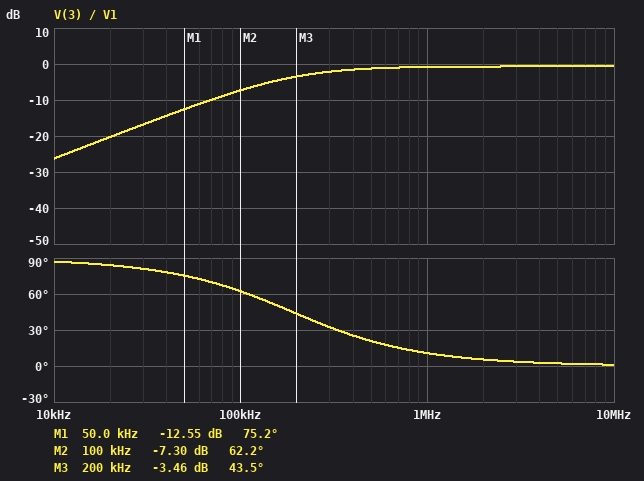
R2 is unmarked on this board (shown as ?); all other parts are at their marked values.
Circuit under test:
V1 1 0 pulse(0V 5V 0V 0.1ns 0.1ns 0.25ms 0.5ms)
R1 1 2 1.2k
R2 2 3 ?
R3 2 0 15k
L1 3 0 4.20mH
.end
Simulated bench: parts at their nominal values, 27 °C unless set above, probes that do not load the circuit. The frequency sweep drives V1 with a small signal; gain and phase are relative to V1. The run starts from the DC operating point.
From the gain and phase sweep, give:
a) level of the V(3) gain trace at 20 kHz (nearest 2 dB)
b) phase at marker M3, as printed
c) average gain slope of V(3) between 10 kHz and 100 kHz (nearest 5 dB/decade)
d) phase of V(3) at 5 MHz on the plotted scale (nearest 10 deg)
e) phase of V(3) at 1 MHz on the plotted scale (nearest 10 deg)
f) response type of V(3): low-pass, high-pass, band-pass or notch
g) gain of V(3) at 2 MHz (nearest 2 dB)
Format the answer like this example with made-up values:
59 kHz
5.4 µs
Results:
-20 dB
43.5 deg
20 dB/decade
0 deg
10 deg
high-pass
0 dB
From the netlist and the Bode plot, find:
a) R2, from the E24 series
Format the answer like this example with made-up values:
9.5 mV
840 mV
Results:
3.9 kΩ
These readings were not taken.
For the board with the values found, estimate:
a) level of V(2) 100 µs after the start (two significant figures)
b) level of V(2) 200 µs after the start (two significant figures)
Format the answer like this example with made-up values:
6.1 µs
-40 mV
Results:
3.6 V
3.6 V
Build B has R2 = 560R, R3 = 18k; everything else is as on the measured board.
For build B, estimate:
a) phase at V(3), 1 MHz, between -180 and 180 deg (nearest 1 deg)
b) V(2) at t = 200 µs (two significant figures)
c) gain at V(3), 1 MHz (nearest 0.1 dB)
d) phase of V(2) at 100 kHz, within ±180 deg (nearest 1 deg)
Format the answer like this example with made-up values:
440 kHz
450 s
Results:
4 deg
1.6 V
-0.6 dB
21 deg
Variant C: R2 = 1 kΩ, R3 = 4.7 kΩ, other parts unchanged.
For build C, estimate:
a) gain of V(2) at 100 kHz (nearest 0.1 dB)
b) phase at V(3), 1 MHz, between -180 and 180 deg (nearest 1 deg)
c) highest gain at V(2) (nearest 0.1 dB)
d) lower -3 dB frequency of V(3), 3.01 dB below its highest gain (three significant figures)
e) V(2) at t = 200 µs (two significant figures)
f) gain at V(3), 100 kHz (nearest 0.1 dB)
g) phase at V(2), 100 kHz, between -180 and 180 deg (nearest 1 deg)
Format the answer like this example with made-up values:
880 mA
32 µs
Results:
-3.3 dB
4 deg
-2.0 dB
74.1 kHz
2.0 V
-3.9 dB
16 deg
